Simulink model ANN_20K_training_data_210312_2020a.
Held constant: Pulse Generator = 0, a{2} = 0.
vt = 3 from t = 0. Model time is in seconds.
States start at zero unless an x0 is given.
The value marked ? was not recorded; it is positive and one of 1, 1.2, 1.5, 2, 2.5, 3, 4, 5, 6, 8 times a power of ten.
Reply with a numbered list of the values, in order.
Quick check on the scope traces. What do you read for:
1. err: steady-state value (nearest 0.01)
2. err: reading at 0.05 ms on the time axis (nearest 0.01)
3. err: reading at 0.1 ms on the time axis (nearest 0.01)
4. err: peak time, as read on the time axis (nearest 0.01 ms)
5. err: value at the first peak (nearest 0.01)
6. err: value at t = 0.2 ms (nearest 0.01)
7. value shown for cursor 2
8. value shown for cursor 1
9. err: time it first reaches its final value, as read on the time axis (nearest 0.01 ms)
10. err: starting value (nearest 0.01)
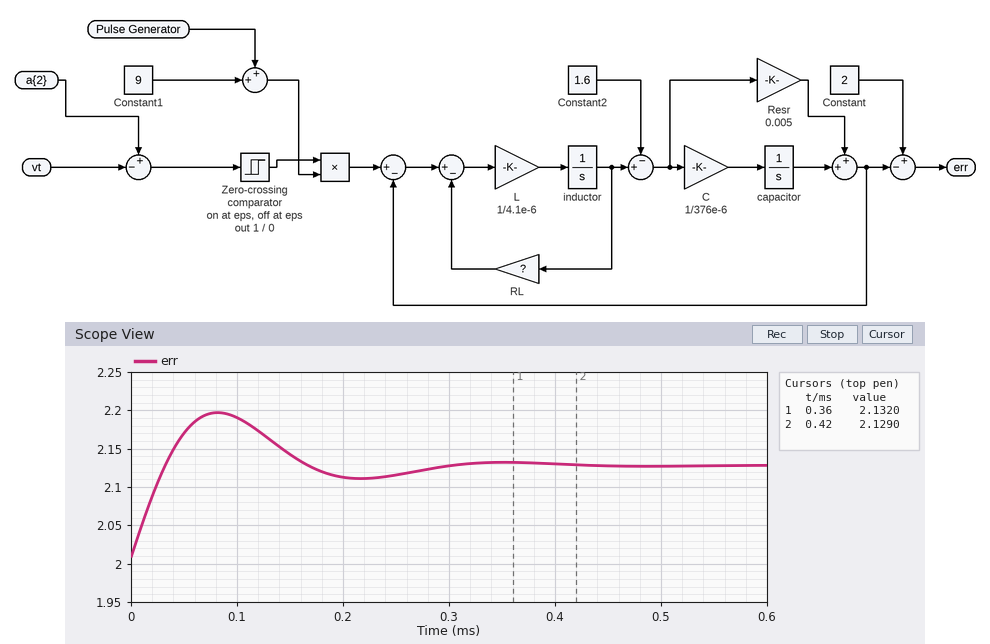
1. 2.13
2. 2.17
3. 2.19
4. 0.08 ms
5. 2.20
6. 2.11
7. 2.1290
8. 2.1320
9. 0.03 ms
10. 2.01
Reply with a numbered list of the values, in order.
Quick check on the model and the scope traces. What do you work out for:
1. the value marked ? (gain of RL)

1. 0.08
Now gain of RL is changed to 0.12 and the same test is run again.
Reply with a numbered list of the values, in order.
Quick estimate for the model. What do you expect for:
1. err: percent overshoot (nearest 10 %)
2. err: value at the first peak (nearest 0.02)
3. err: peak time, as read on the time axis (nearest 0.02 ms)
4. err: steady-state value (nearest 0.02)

1. 20 %
2. 2.22
3. 0.10 ms
4. 2.20
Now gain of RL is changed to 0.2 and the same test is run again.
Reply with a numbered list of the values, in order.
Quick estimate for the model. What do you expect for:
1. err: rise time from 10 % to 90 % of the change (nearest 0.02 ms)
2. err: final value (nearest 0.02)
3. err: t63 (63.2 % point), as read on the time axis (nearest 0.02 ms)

1. 0.12 ms
2. 2.32
3. 0.06 ms
